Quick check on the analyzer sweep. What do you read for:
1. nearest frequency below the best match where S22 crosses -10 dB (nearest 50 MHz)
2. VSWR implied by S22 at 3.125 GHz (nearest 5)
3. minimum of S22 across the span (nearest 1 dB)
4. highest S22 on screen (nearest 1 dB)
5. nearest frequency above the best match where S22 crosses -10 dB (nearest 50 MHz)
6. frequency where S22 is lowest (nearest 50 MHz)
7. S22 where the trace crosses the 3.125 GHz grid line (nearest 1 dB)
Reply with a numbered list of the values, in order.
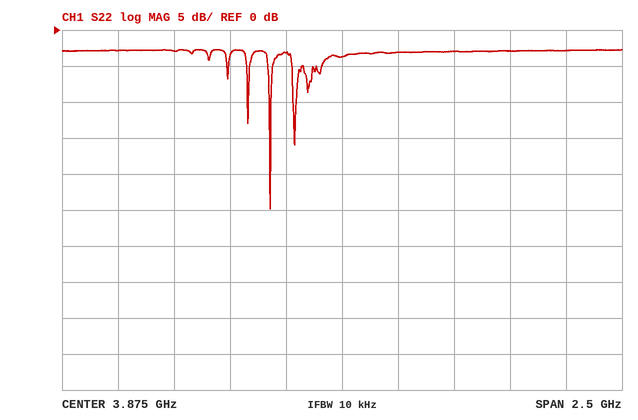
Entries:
1. 3.55 GHz
2. 5
3. -25 dB
4. -3 dB
5. 3.55 GHz
6. 3.55 GHz
7. -3 dB
